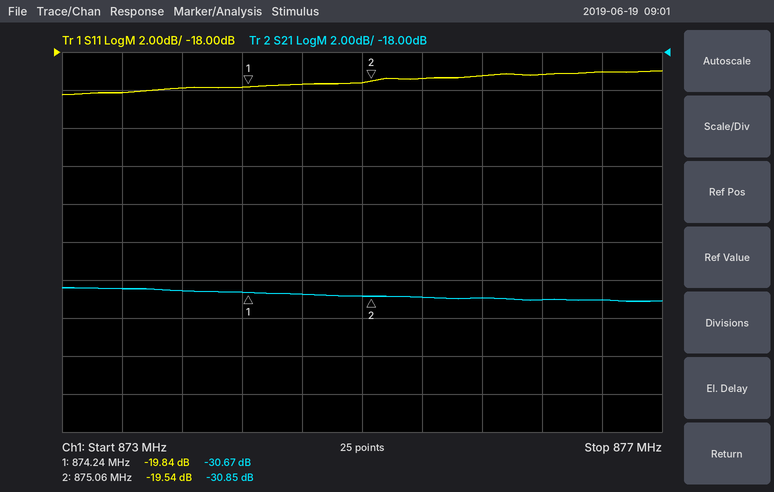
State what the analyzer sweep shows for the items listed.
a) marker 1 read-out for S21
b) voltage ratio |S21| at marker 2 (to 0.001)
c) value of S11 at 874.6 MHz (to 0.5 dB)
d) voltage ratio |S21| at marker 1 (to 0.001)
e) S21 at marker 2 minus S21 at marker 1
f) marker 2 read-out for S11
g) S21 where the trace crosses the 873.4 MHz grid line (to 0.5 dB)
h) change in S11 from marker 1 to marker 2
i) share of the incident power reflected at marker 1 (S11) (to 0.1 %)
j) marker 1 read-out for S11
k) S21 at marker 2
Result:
-30.67 dB
0.029
-19.5 dB
0.029
-0.18 dB
-19.54 dB
-30.5 dB
0.30 dB
1.0 %
-19.84 dB
-30.85 dB
